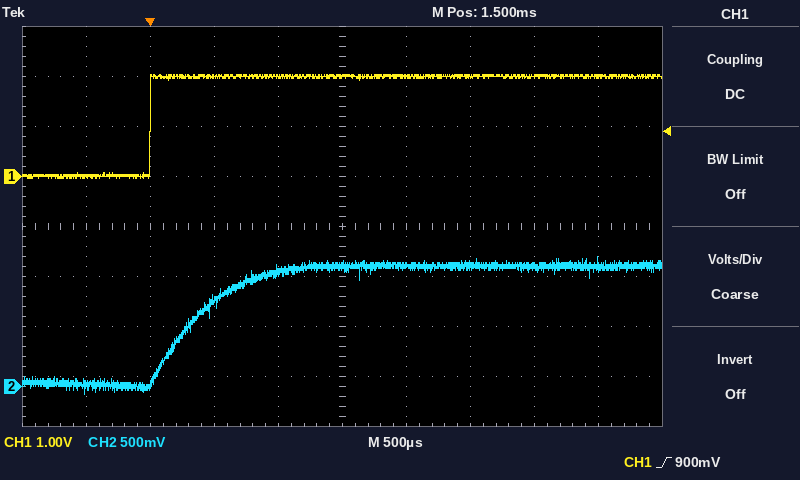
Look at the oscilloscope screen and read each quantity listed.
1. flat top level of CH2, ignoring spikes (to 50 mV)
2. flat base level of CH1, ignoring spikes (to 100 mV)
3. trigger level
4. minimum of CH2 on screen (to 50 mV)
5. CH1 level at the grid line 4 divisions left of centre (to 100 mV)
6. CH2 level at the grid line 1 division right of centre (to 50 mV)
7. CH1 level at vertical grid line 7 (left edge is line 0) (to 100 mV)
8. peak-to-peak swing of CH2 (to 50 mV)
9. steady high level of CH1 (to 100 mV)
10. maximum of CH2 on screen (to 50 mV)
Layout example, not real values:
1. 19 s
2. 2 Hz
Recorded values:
1. 1.20 V
2. 0.0 V
3. 900 mV
4. -100 mV
5. 0.0 V
6. 1.20 V
7. 2.0 V
8. 1.40 V
9. 2.0 V
10. 1.30 V
